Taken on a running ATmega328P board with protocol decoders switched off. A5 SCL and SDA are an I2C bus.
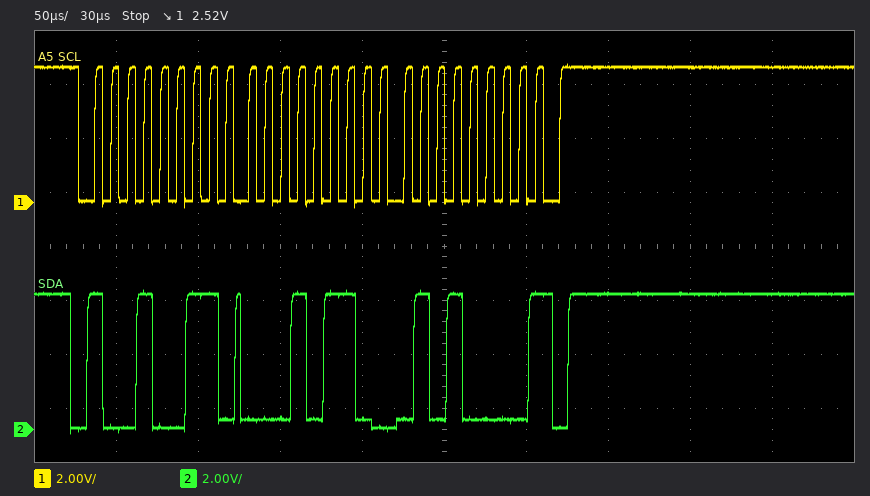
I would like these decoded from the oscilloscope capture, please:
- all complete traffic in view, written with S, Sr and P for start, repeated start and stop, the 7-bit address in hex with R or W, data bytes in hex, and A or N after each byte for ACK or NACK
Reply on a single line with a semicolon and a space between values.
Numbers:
S 49R A 16 A 50 N P
